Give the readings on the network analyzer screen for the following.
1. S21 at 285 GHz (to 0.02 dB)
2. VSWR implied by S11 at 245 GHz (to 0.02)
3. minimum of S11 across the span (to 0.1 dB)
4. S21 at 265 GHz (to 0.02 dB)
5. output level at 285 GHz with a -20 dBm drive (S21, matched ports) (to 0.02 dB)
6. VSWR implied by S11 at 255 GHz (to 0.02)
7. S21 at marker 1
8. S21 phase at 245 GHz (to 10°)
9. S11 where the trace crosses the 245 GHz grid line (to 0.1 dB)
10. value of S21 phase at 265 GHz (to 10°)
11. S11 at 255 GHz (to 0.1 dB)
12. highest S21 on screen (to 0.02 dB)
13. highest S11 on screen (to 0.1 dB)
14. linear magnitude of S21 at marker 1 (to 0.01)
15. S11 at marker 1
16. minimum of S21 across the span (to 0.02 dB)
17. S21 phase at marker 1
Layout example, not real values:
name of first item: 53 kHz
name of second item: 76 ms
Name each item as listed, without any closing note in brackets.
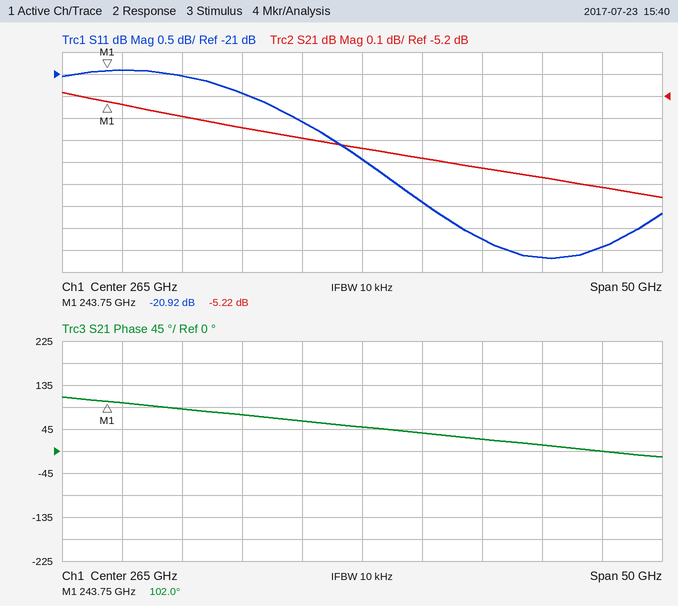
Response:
S21 at 285 GHz: -5.62 dB
VSWR implied by S11 at 245 GHz: 1.20
minimum of S11 across the span: -25.2 dB
S21 at 265 GHz: -5.44 dB
output level at 285 GHz with a -20 dBm drive (S21, matched ports): -25.62 dBm
VSWR implied by S11 at 255 GHz: 1.18
S21 at marker 1: -5.22 dB
S21 phase at 245 GHz: 100°
S11 where the trace crosses the 245 GHz grid line: -20.9 dB
value of S21 phase at 265 GHz: 50°
S11 at 255 GHz: -21.4 dB
highest S21 on screen: -5.18 dB
highest S11 on screen: -20.9 dB
linear magnitude of S21 at marker 1: 0.55
S11 at marker 1: -20.92 dB
minimum of S21 across the span: -5.66 dB
S21 phase at marker 1: 102.0°
